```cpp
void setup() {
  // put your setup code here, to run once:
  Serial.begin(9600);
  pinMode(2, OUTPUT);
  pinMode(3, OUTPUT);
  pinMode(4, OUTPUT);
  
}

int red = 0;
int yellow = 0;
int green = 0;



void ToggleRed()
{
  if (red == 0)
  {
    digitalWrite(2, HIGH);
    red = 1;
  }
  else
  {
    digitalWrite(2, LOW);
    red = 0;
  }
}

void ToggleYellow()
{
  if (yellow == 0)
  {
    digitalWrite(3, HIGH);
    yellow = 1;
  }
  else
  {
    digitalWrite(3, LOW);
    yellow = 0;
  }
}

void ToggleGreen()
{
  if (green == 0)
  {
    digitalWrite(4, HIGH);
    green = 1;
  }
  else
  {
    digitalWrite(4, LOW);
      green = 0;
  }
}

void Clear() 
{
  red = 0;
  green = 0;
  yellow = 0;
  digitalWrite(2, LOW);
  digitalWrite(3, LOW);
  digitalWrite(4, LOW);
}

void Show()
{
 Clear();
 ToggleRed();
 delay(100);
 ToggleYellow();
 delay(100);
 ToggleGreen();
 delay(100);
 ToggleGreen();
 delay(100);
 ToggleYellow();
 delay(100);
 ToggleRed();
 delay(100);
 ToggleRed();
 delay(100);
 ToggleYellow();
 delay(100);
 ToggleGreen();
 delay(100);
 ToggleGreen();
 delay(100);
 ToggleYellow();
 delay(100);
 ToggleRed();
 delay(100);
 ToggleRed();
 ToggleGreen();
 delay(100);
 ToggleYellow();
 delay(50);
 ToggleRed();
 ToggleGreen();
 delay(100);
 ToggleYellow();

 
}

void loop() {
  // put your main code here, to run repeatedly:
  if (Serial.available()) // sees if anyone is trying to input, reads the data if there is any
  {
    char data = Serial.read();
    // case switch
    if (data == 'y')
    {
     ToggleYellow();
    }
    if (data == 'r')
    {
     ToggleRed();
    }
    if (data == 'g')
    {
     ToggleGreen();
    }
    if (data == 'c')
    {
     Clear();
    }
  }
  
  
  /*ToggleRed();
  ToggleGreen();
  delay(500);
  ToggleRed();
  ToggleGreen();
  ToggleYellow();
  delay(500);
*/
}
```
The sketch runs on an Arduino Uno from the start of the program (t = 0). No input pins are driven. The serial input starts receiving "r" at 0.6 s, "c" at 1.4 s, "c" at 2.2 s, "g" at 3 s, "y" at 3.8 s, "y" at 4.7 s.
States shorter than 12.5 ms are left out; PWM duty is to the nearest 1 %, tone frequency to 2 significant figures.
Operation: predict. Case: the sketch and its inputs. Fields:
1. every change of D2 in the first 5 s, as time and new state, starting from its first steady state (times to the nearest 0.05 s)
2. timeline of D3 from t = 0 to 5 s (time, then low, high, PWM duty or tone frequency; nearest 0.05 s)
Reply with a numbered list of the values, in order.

1. 0 s low; 0.6 s high; 1.4 s low
2. 0 s low; 3.8 s high; 4.7 s low
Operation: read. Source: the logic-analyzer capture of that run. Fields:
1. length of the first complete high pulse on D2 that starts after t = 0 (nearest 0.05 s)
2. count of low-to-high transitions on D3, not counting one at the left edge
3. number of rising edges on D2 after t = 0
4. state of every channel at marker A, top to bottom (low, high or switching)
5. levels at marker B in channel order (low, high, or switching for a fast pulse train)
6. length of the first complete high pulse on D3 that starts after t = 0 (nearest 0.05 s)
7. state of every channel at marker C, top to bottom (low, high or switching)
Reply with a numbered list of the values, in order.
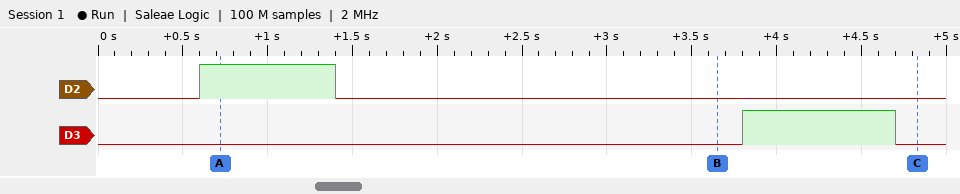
1. 0.80 s
2. 1
3. 1
4. D2 high, D3 low
5. D2 low, D3 low
6. 0.90 s
7. D2 low, D3 low
